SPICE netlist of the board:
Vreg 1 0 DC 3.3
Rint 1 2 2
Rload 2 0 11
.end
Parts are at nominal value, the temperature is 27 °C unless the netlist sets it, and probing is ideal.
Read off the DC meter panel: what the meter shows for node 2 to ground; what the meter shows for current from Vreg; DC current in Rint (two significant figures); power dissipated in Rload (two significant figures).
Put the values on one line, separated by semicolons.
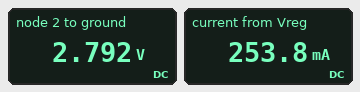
2.792 V; 253.8 mA; 250 mA; 710 mW
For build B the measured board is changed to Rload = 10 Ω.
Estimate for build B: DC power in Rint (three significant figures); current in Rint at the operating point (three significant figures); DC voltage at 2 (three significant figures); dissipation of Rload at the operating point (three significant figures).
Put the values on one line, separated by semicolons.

151 mW; 275 mA; 2.75 V; 756 mW
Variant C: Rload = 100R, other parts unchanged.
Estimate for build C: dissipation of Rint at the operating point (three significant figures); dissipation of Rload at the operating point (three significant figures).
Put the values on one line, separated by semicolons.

2.09 mW; 105 mW
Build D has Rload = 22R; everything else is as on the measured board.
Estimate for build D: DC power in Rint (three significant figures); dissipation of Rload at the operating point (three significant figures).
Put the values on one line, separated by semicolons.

37.8 mW; 416 mW
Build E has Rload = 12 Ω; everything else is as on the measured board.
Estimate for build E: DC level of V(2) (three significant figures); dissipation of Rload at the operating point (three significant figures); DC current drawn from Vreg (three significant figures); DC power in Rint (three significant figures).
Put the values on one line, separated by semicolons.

2.83 V; 667 mW; 236 mA; 111 mW
